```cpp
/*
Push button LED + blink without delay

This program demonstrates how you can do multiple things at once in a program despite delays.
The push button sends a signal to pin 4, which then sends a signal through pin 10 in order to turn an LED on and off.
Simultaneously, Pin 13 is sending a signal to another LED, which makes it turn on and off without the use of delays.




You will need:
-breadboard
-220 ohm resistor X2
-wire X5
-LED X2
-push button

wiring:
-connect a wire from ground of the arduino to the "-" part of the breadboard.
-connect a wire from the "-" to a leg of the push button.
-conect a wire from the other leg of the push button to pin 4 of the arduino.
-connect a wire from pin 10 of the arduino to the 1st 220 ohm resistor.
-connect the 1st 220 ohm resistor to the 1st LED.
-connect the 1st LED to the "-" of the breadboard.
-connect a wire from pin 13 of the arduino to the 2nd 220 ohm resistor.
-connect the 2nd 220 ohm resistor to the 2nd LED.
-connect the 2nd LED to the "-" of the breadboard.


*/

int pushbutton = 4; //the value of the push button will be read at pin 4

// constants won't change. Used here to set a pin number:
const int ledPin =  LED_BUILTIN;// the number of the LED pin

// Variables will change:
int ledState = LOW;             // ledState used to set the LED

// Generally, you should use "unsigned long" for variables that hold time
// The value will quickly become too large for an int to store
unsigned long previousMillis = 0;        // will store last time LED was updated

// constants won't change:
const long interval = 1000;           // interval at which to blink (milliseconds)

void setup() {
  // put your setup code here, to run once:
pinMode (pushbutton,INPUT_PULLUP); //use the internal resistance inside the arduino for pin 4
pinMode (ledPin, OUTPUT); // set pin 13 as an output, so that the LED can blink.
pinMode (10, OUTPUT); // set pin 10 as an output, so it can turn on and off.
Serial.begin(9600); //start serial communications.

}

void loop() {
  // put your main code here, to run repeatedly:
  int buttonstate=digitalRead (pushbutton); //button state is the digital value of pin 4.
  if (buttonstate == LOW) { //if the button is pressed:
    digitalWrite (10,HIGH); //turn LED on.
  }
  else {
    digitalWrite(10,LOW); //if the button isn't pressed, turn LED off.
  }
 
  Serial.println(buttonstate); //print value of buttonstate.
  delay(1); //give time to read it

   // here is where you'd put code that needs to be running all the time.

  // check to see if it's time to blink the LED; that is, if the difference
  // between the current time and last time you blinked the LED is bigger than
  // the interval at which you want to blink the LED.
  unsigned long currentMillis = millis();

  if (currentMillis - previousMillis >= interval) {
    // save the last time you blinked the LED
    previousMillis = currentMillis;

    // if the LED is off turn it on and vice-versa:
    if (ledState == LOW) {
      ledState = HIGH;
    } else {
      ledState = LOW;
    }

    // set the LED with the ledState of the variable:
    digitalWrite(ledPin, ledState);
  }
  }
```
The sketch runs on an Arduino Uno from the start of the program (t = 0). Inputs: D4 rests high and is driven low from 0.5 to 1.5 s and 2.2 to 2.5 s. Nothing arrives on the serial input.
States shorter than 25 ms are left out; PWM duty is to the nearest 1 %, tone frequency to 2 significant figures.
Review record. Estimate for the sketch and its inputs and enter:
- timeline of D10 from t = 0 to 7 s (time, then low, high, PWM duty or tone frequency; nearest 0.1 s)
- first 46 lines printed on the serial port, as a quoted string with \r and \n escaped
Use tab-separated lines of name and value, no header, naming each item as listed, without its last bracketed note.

timeline of D10 from t = 0 to 7 s	0 s low; 0.5 s high; 1.5 s low; 2.2 s high; 2.5 s low
first 46 lines printed on the serial port, as a quoted string with \r and \n escaped	"1\r\n1\r\n1\r\n1\r\n1\r\n1\r\n1\r\n1\r\n1\r\n1\r\n1\r\n1\r\n1\r\n1\r\n1\r\n1\r\n1\r\n1\r\n1\r\n1\r\n1\r\n1\r\n1\r\n1\r\n1\r\n1\r\n1\r\n1\r\n1\r\n1\r\n1\r\n1\r\n1\r\n1\r\n1\r\n1\r\n1\r\n1\r\n1\r\n1\r\n1\r\n1\r\n1\r\n1\r\n1\r\n1\r\n"
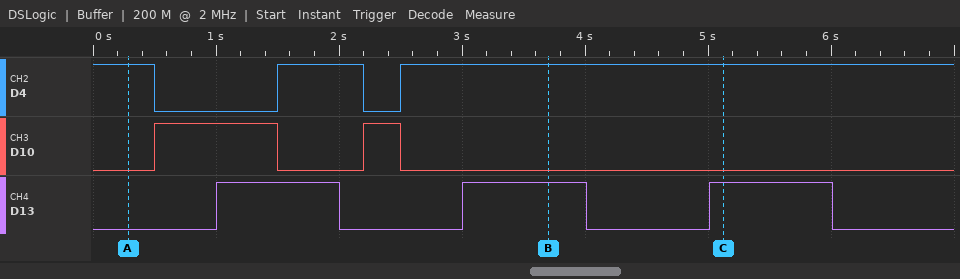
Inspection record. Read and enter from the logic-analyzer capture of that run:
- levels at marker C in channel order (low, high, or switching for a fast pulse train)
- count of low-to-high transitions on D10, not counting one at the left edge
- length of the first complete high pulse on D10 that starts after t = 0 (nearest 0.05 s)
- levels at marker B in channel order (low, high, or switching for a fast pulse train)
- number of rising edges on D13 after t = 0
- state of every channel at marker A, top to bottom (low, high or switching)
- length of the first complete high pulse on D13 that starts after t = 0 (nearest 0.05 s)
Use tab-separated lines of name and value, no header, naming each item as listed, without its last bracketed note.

levels at marker C in channel order	D4 high, D10 low, D13 high
count of low-to-high transitions on D10, not counting one at the left edge	2
length of the first complete high pulse on D10 that starts after t = 0	1.00 s
levels at marker B in channel order	D4 high, D10 low, D13 high
number of rising edges on D13 after t = 0	3
state of every channel at marker A, top to bottom	D4 high, D10 low, D13 low
length of the first complete high pulse on D13 that starts after t = 0	1.00 s
